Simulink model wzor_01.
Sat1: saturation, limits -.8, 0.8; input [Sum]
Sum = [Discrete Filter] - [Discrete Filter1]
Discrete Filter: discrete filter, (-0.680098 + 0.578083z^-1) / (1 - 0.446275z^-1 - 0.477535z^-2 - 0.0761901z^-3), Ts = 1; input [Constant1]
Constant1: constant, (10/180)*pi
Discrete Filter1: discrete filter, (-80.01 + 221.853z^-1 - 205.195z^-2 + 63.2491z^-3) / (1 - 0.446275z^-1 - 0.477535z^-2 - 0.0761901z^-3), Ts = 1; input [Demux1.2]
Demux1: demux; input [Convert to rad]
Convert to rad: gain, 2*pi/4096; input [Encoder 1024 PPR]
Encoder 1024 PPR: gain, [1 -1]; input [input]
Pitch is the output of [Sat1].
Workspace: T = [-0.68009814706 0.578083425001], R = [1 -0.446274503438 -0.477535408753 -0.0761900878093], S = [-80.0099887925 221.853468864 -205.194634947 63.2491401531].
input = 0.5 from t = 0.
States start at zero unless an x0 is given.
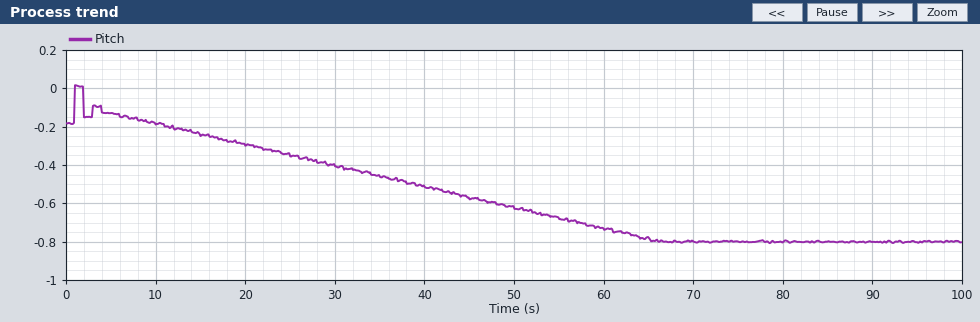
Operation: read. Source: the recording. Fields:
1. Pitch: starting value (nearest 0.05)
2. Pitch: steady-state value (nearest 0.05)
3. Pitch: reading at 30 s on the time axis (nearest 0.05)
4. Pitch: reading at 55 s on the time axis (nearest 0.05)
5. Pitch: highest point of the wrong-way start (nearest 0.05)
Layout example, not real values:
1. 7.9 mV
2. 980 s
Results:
1. -0.20
2. -0.80
3. -0.40
4. -0.70
5. 0.00
